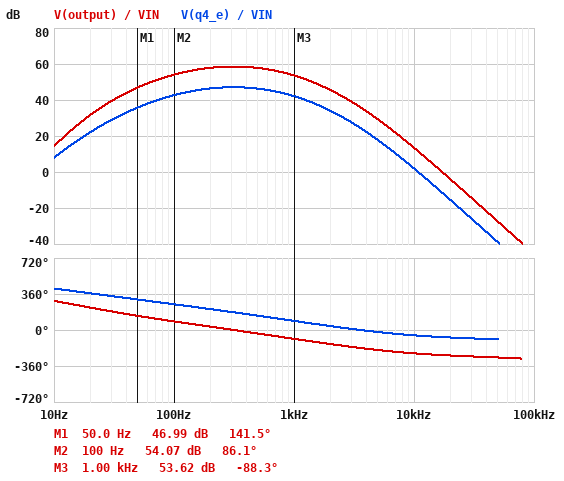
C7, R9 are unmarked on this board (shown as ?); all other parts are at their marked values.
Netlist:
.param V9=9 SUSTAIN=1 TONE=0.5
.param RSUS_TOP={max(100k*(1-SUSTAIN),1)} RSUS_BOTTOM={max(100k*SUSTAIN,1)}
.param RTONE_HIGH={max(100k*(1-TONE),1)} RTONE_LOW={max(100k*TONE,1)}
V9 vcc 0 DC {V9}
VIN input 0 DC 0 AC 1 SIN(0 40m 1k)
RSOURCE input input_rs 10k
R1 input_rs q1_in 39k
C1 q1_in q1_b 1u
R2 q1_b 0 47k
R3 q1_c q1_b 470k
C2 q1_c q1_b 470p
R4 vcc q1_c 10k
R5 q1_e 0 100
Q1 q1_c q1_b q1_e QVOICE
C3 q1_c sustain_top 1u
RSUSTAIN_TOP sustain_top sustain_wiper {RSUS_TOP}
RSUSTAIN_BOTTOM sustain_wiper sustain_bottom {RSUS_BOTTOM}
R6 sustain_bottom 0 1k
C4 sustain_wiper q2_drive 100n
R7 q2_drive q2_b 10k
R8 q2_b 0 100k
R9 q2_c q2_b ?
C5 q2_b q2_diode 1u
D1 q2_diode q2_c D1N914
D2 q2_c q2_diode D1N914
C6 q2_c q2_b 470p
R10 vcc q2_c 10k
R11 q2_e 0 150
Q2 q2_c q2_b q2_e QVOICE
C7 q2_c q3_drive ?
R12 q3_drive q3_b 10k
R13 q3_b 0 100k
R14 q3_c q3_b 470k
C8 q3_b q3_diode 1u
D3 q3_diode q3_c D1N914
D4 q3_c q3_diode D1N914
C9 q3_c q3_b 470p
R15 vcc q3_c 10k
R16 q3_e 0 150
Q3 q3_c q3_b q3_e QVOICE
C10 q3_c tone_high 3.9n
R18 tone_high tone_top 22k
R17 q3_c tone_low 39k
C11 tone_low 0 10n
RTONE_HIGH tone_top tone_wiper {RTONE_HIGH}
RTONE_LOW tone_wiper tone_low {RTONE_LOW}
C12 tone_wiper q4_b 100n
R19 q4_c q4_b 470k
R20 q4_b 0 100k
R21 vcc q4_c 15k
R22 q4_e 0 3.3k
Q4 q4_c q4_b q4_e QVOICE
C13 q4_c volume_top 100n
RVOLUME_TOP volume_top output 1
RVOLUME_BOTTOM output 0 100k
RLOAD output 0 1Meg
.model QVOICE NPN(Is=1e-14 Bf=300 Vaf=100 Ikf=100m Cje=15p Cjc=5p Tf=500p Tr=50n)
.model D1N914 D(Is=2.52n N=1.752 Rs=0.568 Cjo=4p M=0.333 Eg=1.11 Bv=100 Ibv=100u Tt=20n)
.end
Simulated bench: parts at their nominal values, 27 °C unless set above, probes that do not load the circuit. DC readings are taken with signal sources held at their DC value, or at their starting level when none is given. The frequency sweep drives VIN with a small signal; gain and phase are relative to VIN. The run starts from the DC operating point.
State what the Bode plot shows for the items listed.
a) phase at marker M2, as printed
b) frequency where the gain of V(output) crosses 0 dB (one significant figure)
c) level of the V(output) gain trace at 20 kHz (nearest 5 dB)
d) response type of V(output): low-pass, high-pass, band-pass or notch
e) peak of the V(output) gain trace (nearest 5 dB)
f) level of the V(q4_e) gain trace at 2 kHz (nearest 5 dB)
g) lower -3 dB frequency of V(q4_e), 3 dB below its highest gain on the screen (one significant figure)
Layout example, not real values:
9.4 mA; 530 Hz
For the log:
86.1 deg; 20 kHz; -5 dB; band-pass; 60 dB; 35 dB; 100 Hz
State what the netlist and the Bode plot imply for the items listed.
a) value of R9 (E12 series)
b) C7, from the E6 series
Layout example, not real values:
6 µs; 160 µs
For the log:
1.2 MΩ; 33 nF
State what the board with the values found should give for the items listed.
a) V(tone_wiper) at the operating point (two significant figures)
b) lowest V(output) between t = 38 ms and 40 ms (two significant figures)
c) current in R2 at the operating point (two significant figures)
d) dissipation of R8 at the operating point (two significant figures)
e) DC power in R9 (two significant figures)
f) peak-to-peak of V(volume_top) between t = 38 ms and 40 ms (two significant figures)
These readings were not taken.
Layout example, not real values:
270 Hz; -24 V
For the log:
4.6 V; -450 mV; 13 µA; 3.6 µW; 47 µW; 870 mV
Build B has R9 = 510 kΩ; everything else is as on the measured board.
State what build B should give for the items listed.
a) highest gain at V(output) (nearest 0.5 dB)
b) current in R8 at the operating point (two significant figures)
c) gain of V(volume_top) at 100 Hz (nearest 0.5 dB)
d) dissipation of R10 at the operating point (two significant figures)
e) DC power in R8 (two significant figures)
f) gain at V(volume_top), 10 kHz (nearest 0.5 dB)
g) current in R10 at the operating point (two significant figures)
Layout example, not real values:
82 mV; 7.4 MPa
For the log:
61.0 dB; 6.9 µA; 55.0 dB; 1.7 mW; 4.8 µW; 14.5 dB; 410 µA
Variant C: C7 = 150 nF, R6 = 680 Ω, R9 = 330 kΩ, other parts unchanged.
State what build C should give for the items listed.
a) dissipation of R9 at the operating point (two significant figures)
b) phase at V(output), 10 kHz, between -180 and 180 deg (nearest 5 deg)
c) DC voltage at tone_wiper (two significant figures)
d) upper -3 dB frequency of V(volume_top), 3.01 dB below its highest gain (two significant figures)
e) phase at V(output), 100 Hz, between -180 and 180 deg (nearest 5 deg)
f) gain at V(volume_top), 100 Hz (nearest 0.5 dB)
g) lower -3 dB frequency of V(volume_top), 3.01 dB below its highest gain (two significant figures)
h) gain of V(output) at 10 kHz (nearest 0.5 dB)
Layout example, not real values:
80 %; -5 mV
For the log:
26 µW; 120 deg; 4.6 V; 710 Hz; 70 deg; 59.5 dB; 83 Hz; 14.5 dB
